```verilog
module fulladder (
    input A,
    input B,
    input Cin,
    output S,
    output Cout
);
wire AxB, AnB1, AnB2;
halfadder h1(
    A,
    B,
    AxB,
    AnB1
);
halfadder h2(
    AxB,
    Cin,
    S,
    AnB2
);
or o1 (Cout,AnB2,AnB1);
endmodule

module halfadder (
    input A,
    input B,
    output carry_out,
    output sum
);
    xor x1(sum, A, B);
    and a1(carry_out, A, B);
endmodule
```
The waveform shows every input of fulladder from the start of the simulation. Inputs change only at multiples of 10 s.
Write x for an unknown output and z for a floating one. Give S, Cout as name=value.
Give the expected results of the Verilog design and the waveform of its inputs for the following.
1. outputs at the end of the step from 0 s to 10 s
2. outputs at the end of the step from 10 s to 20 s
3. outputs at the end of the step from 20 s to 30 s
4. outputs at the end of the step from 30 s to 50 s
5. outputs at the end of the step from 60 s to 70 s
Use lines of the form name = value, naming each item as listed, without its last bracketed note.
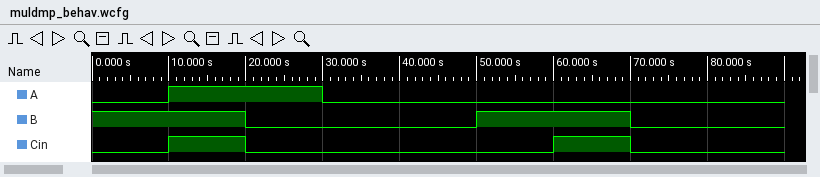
outputs at the end of the step from 0 s to 10 s = S=0, Cout=1
outputs at the end of the step from 10 s to 20 s = S=1, Cout=0
outputs at the end of the step from 20 s to 30 s = S=0, Cout=1
outputs at the end of the step from 30 s to 50 s = S=0, Cout=0
outputs at the end of the step from 60 s to 70 s = S=0, Cout=1
